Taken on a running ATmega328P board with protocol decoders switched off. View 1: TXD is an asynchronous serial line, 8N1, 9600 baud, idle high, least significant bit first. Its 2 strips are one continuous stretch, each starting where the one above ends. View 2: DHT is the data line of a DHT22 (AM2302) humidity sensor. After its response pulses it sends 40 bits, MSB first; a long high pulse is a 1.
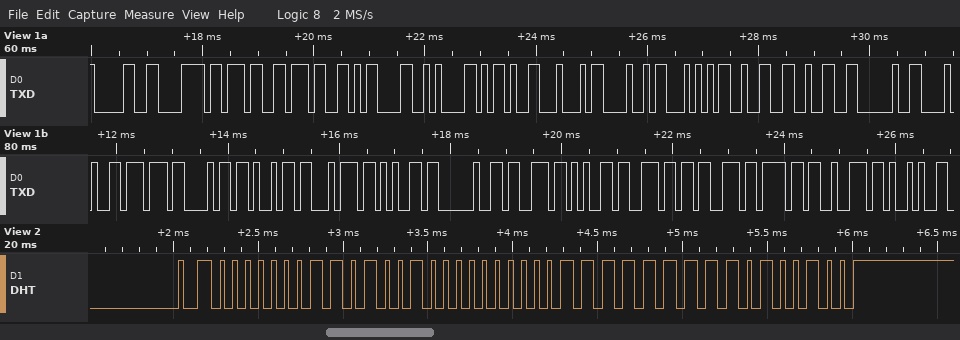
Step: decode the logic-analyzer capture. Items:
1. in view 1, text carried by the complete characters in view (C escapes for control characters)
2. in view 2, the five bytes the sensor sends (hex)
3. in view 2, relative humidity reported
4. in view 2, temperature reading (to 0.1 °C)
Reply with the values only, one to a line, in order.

"0x77\r\n-DHT22 (white sensor)"
01 A4 00 FF A4
42.0 %
25.5 °C
